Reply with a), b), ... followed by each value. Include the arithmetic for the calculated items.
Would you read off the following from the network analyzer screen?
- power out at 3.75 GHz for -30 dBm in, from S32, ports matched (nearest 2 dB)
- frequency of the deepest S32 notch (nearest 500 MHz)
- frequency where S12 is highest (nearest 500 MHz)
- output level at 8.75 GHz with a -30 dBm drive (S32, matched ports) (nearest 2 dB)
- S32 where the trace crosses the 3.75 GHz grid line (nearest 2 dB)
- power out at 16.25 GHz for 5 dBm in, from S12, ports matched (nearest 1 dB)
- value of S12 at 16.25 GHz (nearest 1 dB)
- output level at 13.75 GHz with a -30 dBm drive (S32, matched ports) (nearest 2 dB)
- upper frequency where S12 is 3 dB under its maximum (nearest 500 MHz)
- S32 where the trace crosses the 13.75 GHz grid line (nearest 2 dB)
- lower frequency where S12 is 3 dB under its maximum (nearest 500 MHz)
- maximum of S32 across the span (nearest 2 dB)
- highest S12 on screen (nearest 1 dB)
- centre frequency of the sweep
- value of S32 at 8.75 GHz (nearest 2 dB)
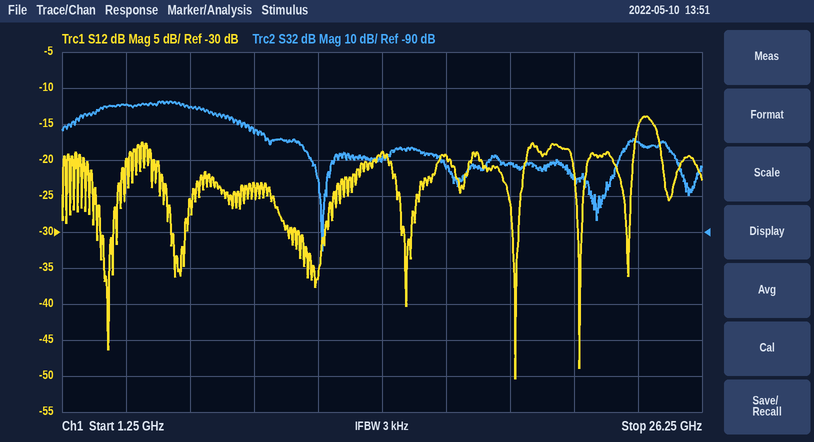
a) -30 dBm + (-54 dB) = -84 dBm
b) 11.5 GHz
c) 24.0 GHz
d) -30 dBm + (-62 dB) = -92 dBm
e) -54 dB
f) 5 dBm + (-19 dB) = -14 dBm
g) -19 dB
h) -30 dBm + (-70 dB) = -100 dBm
i) 24.5 GHz
j) -70 dB
k) 23.5 GHz
l) -54 dB
m) -14 dB
n) 13.75 GHz
o) -62 dB
